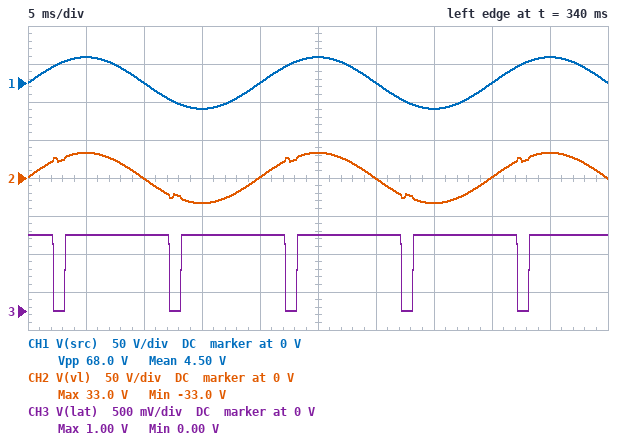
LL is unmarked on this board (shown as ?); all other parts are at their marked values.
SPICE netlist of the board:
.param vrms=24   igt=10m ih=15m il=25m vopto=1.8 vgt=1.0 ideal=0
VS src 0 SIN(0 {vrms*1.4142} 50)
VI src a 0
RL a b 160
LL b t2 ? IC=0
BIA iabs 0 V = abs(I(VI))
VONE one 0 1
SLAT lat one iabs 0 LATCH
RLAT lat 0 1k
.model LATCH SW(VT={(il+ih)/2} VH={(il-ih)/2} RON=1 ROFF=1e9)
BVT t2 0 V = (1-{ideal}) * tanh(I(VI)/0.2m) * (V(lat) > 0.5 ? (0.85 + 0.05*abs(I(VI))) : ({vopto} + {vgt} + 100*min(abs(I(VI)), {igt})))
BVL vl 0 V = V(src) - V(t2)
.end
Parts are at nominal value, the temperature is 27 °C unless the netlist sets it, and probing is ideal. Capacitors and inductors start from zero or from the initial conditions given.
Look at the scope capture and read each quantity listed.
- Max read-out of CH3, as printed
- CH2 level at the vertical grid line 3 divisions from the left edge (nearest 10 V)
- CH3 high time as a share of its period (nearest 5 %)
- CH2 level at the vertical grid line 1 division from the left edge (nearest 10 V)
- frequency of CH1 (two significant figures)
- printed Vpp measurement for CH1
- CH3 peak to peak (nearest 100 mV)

1.00 V
-30 V
90 %
30 V
50 Hz
68.0 V
1.0 V
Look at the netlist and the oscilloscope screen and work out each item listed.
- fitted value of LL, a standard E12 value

560 mH
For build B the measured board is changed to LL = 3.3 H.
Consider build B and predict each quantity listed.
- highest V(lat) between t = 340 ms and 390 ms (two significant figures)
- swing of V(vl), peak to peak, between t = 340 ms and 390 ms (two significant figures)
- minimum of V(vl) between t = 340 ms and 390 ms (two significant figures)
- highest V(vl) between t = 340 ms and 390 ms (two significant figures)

1.0 V
71 V
-36 V
36 V
